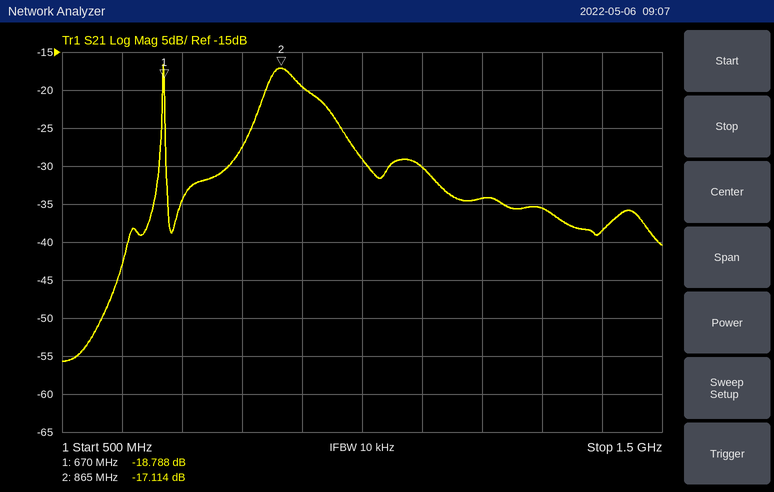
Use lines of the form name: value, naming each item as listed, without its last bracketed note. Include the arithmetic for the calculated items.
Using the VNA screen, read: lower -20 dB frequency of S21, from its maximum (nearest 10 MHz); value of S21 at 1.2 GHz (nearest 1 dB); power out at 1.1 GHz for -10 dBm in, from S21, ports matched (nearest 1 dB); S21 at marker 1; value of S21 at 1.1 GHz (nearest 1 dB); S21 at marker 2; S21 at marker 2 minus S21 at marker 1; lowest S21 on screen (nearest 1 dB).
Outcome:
lower -20 dB frequency of S21, from its maximum: 650 MHz
value of S21 at 1.2 GHz: -34 dB
power out at 1.1 GHz for -10 dBm in, from S21, ports matched: -10 dBm + (-30 dB) = -40 dBm
S21 at marker 1: -18.788 dB
value of S21 at 1.1 GHz: -30 dB
S21 at marker 2: -17.114 dB
S21 at marker 2 minus S21 at marker 1: -17.114 − (-18.788) = 1.674 dB
lowest S21 on screen: -56 dB
